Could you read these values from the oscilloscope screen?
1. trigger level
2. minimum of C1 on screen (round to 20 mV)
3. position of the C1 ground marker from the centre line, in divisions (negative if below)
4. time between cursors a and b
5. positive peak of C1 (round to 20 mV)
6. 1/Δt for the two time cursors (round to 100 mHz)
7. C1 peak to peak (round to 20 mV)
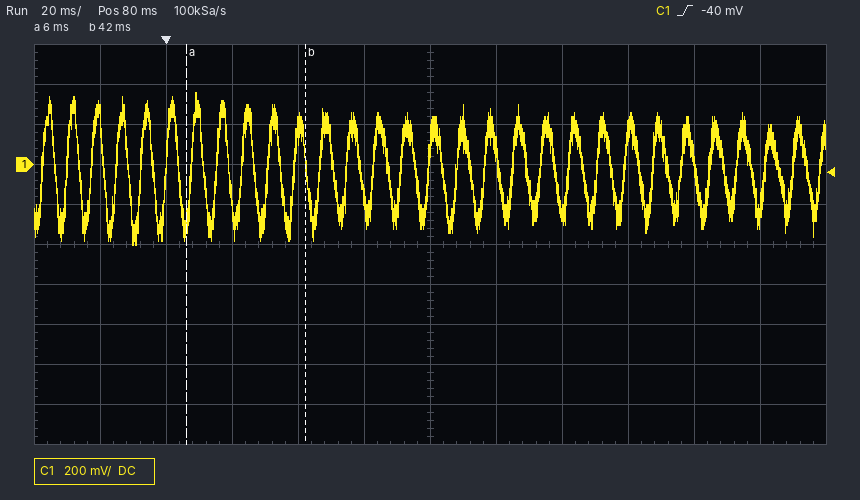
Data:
-40 mV
-400 mV
+2.0 div
36 ms
360 mV
27.8 Hz
760 mV
